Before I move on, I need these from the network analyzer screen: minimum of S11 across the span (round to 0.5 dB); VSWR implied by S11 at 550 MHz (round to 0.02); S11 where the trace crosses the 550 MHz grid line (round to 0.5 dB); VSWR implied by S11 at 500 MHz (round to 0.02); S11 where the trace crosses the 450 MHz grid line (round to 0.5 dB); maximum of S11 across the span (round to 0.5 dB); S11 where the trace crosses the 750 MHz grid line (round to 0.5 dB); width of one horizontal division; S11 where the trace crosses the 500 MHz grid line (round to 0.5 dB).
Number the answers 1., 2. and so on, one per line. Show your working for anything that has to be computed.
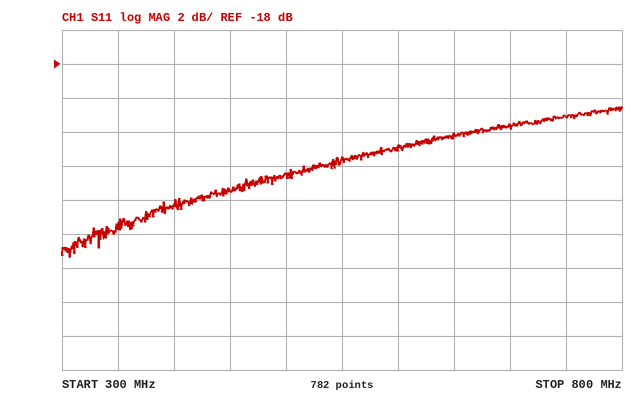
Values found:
1. -29.5 dB
2. |Γ| = 10^(-23.5/20) = 0.0668; VSWR = (1 + 0.0668)/(1 − 0.0668) ≈ 1.14
3. -23.5 dB
4. |Γ| = 10^(-24.5/20) = 0.0596; VSWR = (1 + 0.0596)/(1 − 0.0596) ≈ 1.13, so 1.12 to the nearest 0.02
5. -25.5 dB
6. -20.5 dB
7. -21.0 dB
8. 50 MHz
9. -24.5 dB
